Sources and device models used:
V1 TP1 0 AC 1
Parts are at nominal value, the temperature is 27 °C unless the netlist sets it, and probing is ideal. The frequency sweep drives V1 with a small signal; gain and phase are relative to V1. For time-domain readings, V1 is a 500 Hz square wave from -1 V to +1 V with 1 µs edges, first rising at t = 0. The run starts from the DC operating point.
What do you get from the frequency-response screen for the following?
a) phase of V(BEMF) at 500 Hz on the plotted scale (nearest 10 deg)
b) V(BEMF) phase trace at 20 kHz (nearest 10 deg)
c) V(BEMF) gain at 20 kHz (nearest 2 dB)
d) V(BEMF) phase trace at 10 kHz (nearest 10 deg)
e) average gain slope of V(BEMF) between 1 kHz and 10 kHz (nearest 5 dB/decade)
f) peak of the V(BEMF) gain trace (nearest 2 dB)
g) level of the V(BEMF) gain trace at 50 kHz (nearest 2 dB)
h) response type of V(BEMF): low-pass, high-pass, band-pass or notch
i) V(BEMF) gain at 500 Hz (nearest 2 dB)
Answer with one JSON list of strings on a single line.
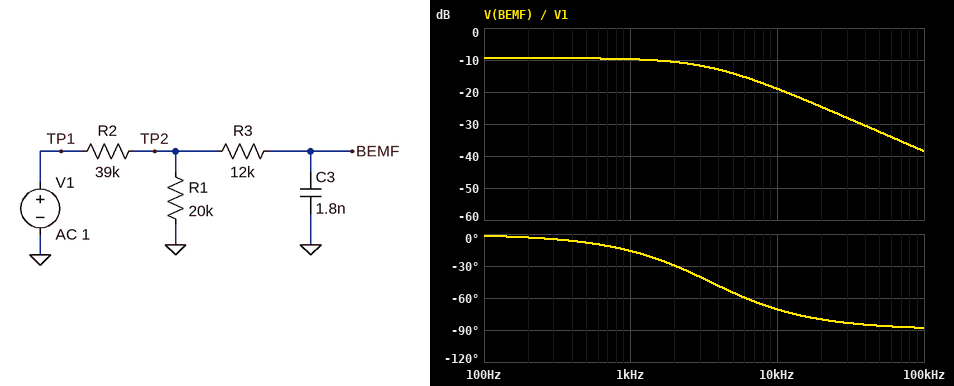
["-10 deg", "-80 deg", "-24 dB", "-70 deg", "-10 dB/decade", "-10 dB", "-32 dB", "low-pass", "-10 dB"]
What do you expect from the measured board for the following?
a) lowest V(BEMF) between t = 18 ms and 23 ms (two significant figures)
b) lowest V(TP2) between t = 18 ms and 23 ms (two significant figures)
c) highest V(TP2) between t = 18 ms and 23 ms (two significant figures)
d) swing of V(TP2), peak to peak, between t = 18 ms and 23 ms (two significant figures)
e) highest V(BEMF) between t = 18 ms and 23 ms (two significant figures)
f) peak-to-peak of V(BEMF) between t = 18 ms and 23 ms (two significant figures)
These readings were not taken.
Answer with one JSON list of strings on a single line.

["-340 mV", "-340 mV", "340 mV", "680 mV", "340 mV", "680 mV"]
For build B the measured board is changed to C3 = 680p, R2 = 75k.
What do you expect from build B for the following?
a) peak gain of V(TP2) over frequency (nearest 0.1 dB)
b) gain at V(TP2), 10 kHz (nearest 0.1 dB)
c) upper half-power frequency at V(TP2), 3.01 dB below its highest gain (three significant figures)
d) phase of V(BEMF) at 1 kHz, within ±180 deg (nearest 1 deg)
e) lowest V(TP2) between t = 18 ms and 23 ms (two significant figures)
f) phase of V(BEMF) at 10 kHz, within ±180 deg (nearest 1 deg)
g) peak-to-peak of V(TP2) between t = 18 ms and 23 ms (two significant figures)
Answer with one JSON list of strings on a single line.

["-13.5 dB", "-16.3 dB", "10.6 kHz", "-7 deg", "-210 mV", "-50 deg", "420 mV"]
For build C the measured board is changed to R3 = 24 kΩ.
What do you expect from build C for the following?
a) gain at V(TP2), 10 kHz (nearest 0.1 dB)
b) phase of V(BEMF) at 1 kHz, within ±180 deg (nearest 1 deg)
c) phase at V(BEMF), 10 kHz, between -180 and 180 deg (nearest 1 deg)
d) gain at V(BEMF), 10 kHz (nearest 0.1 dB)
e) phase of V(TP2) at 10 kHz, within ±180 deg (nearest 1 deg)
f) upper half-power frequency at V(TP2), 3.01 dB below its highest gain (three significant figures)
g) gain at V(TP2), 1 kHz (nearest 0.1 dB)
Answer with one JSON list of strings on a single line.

["-12.9 dB", "-23 deg", "-77 deg", "-22.1 dB", "-7 deg", "5.79 kHz", "-9.8 dB"]
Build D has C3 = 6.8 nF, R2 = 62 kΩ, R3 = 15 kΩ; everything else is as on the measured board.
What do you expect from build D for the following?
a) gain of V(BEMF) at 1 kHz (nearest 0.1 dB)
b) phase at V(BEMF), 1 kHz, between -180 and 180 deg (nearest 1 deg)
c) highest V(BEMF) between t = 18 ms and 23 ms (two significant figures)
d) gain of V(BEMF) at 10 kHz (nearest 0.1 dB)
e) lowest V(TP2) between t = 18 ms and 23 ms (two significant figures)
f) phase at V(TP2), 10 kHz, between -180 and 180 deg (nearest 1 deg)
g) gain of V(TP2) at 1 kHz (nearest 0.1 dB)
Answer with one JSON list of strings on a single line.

["-16.5 dB", "-52 deg", "240 mV", "-34.5 dB", "-240 mV", "-4 deg", "-15.0 dB"]
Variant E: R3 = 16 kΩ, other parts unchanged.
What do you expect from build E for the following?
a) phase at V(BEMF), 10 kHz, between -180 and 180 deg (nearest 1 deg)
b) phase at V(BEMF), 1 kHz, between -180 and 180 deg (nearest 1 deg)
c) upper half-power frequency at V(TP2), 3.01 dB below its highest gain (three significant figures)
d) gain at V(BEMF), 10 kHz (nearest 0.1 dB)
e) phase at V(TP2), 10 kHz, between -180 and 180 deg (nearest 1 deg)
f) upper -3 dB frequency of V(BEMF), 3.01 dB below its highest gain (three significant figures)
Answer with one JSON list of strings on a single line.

["-73 deg", "-18 deg", "4.78 kHz", "-20.2 dB", "-12 deg", "3.03 kHz"]
